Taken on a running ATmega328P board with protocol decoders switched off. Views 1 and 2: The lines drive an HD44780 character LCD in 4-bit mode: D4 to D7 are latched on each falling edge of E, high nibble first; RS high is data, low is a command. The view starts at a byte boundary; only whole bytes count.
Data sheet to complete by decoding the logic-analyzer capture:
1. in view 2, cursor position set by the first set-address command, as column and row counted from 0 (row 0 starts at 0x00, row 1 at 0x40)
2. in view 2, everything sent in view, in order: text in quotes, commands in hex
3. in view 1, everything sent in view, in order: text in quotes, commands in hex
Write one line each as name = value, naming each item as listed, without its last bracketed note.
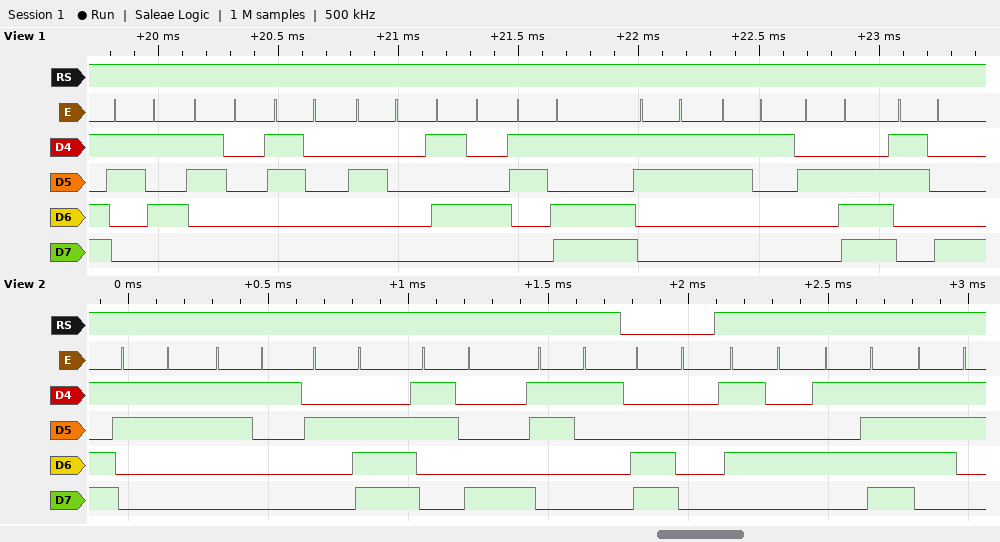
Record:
in view 2, cursor position set by the first set-address command, as column and row counted from 0 = column 0, row 1
in view 2, everything sent in view, in order: text in quotes, commands in hex = "31.81" 0xC0 "T_s"
in view 1, everything sent in view, in order: text in quotes, commands in hex = "500 T=31.8"
